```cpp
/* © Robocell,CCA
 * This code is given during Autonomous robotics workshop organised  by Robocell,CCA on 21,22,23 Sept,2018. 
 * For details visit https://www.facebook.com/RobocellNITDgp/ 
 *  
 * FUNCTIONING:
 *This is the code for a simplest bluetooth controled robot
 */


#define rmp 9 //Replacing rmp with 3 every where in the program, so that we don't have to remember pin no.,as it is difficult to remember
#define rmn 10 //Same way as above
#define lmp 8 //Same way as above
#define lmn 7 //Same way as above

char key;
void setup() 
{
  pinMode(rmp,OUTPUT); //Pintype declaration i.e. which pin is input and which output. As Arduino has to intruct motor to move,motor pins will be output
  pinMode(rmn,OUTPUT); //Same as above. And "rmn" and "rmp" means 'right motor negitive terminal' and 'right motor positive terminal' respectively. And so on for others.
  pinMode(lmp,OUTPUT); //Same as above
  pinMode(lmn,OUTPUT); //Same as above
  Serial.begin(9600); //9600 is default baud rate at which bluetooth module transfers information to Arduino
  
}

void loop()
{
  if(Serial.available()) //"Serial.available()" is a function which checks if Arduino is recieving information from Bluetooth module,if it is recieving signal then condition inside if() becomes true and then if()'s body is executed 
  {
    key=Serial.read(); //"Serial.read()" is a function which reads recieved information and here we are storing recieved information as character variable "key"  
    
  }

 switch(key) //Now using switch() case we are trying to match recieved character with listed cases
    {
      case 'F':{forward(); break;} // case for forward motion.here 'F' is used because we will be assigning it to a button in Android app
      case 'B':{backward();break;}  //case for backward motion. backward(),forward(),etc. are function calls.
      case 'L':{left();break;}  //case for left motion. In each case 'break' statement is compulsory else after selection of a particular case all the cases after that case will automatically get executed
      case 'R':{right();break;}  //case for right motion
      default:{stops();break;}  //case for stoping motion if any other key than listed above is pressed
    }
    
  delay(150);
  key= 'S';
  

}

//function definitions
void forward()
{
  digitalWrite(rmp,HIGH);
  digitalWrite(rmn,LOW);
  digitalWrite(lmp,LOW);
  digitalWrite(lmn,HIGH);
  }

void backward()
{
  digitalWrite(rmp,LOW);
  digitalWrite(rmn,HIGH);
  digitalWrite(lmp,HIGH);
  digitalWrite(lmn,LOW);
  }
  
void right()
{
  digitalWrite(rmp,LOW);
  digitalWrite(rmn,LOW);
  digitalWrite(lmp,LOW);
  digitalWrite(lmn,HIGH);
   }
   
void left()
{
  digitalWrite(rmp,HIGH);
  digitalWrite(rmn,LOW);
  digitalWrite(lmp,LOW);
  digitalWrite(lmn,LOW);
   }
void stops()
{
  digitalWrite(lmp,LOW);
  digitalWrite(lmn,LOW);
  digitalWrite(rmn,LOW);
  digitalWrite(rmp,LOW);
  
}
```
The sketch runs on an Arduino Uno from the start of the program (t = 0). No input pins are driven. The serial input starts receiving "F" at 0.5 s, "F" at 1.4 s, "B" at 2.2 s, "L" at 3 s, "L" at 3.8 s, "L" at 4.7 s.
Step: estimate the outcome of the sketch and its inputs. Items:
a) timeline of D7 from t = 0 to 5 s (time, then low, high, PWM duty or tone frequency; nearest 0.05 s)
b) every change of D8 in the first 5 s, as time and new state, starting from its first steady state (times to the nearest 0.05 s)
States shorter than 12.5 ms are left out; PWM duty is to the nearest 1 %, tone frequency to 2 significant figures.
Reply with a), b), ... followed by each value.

a) 0 s low; 0.6 s high; 0.75 s low; 1.5 s high; 1.65 s low
b) 0 s low; 2.25 s high; 2.4 s low
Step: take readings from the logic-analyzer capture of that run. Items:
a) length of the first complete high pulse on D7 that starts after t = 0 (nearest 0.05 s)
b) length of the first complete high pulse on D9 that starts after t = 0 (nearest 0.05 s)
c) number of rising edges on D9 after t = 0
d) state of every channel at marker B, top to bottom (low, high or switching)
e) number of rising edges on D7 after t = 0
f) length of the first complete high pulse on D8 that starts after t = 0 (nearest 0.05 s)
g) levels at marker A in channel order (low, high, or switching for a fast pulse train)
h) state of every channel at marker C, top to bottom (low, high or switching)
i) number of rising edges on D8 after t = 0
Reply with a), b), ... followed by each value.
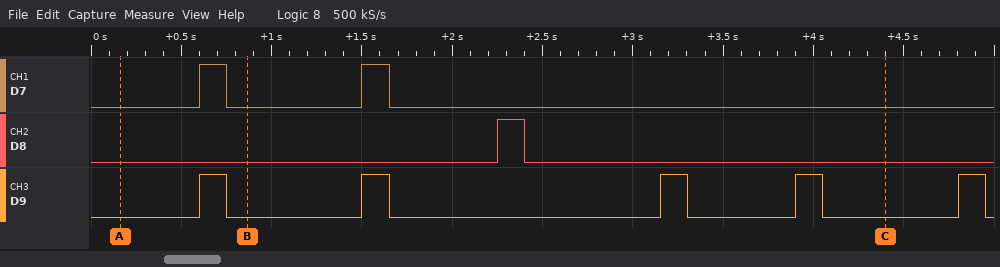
a) 0.15 s
b) 0.15 s
c) 5
d) D7 low, D8 low, D9 low
e) 2
f) 0.15 s
g) D7 low, D8 low, D9 low
h) D7 low, D8 low, D9 low
i) 1
